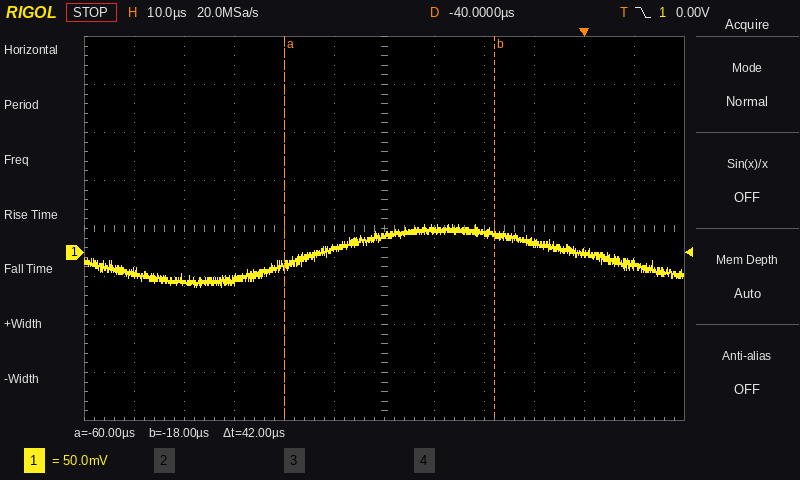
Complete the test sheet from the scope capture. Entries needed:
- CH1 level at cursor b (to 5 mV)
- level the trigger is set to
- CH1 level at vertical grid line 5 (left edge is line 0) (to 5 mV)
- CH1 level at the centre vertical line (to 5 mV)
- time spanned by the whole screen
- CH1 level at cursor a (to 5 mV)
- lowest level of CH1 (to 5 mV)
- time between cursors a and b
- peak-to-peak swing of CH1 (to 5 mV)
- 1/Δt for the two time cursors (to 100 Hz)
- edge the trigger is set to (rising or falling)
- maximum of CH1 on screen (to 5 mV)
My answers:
20 mV
0.00 V
5 mV
20 mV
120 µs
-15 mV
-35 mV
42 µs
65 mV
23.8 kHz
falling
30 mV
